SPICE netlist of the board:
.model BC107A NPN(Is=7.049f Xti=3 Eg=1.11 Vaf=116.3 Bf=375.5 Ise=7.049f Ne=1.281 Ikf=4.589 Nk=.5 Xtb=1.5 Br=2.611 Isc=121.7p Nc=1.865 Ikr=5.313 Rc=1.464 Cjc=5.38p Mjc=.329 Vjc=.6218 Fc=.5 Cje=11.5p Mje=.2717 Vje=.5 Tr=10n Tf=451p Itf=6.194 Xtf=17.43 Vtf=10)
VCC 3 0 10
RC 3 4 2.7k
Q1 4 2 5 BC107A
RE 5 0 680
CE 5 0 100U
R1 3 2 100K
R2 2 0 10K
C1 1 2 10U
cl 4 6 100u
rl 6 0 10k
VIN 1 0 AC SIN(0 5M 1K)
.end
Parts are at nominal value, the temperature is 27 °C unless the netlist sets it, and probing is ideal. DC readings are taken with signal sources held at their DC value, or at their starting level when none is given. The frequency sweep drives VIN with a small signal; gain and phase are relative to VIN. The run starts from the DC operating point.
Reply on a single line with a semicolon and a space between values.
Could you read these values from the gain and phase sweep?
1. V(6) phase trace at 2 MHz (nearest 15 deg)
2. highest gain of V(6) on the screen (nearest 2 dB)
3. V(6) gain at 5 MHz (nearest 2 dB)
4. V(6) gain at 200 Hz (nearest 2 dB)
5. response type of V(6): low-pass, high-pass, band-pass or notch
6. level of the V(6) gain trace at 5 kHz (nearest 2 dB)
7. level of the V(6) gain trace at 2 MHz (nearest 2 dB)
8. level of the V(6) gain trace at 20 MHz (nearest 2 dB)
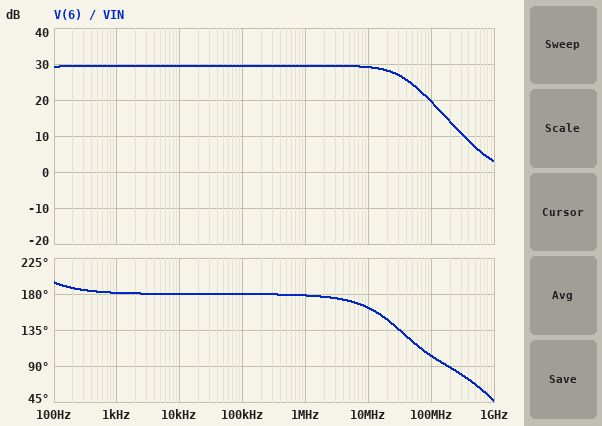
180 deg; 30 dB; 30 dB; 30 dB; low-pass; 30 dB; 30 dB; 28 dB
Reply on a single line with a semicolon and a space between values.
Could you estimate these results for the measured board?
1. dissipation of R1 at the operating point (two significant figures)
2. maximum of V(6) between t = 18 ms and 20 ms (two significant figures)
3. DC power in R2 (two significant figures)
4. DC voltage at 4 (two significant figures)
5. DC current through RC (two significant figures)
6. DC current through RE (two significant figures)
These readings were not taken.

830 µW; 140 mV; 79 µW; 9.0 V; 370 µA; 370 µA
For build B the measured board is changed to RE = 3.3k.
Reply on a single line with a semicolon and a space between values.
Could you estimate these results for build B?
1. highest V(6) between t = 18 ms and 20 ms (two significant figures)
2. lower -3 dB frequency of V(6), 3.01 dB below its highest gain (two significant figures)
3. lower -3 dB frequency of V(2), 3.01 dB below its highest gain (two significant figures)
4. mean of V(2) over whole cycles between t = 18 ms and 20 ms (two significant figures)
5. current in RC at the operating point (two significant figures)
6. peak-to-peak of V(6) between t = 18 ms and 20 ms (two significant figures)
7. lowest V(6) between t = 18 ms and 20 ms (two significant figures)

35 mV; 6.9 Hz; 1.9 Hz; 900 mV; 91 µA; 75 mV; -40 mV
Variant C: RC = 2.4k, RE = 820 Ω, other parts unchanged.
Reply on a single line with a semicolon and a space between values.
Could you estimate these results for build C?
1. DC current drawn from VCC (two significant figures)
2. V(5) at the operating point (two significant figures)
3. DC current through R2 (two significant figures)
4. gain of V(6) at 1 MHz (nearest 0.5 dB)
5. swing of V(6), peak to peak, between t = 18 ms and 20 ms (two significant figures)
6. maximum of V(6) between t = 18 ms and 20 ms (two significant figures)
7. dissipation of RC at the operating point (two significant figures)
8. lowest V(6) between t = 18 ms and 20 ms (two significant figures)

400 µA; 260 mV; 89 µA; 27.5 dB; 230 mV; 110 mV; 230 µW; -120 mV
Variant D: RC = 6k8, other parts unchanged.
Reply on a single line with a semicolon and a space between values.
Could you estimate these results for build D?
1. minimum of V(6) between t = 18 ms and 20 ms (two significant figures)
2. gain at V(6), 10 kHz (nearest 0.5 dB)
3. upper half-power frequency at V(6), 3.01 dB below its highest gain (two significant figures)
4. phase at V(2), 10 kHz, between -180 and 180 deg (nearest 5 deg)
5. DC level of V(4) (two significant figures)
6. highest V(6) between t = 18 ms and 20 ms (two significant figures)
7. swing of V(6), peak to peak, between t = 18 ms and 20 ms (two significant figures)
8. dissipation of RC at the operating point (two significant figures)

-300 mV; 35.0 dB; 17 MHz; 0 deg; 7.5 V; 270 mV; 560 mV; 910 µW
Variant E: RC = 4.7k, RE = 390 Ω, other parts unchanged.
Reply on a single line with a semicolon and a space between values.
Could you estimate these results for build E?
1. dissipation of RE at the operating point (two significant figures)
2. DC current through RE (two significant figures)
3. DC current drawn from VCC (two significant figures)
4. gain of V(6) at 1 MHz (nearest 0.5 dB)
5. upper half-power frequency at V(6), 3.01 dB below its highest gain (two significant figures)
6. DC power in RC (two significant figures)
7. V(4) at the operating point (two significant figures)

130 µW; 580 µA; 670 µA; 37.0 dB; 21 MHz; 1.6 mW; 7.3 V
